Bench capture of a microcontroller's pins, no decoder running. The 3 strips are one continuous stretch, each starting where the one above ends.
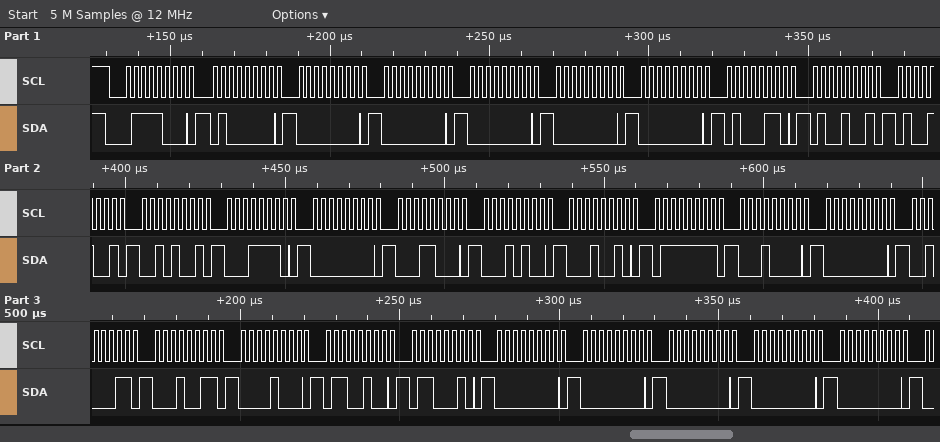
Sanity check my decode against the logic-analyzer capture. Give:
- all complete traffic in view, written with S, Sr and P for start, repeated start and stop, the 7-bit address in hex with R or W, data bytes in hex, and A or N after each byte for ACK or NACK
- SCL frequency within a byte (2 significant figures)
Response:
S 3CW A 40 A 00 A 00 A 00 A 00 A 00 A 46 A 49 A 49 A 29 A 1E A 00 A 18 A 14 A 12 A 7F A 10 A 00 A 23 A 13 A 08 A 64 A 62 A 00 A 00 A 00 A 00 A 00 A
400 kHz
